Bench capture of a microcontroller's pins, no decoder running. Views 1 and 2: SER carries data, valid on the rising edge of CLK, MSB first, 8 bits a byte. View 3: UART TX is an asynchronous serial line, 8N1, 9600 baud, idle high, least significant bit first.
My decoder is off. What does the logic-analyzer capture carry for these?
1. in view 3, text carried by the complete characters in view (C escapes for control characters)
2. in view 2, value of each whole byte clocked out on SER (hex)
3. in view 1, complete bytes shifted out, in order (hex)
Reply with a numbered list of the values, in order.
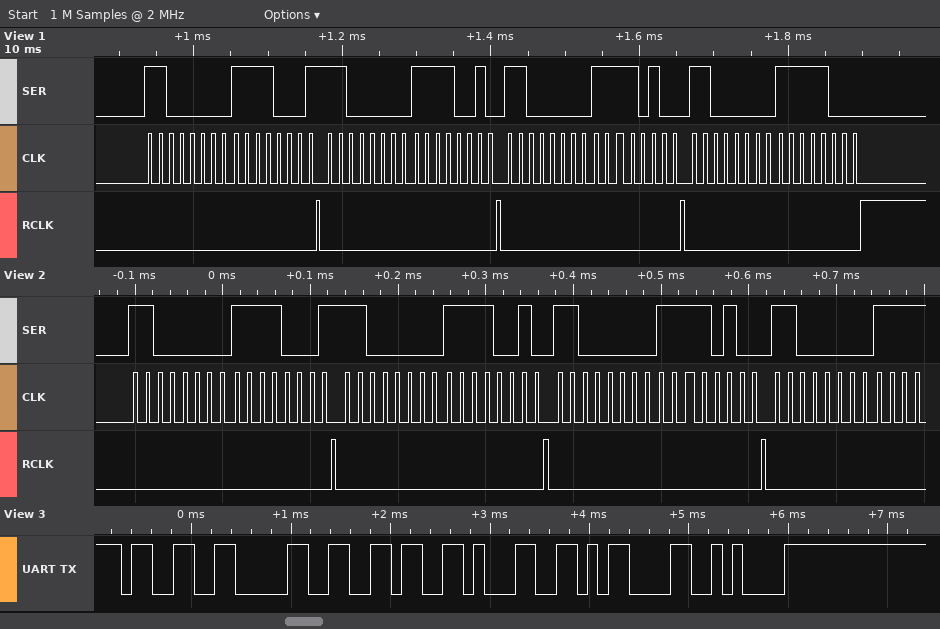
1. "3061\r\n"
2. C0 F1 C0 F2 C0 F4 C0
3. C0 F1 C0 F2 C0 F4 C0 F8
